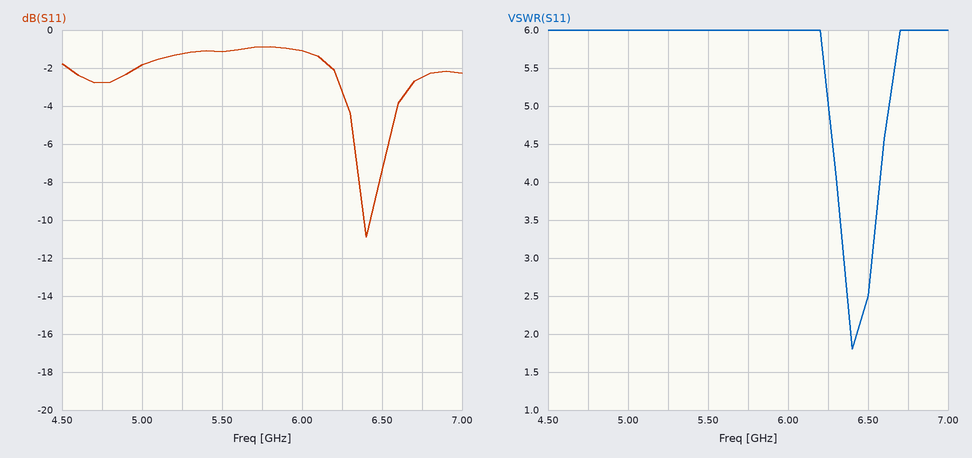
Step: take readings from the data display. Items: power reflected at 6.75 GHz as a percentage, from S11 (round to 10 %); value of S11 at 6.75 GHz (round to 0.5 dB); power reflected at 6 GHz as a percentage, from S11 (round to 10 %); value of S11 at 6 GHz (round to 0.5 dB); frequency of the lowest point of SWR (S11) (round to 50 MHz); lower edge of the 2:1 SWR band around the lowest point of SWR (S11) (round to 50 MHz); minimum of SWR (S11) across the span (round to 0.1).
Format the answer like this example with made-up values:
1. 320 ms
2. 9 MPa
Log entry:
1. 60 %
2. -2.5 dB
3. 80 %
4. -1.0 dB
5. 6.40 GHz
6. 6.40 GHz
7. 1.8
